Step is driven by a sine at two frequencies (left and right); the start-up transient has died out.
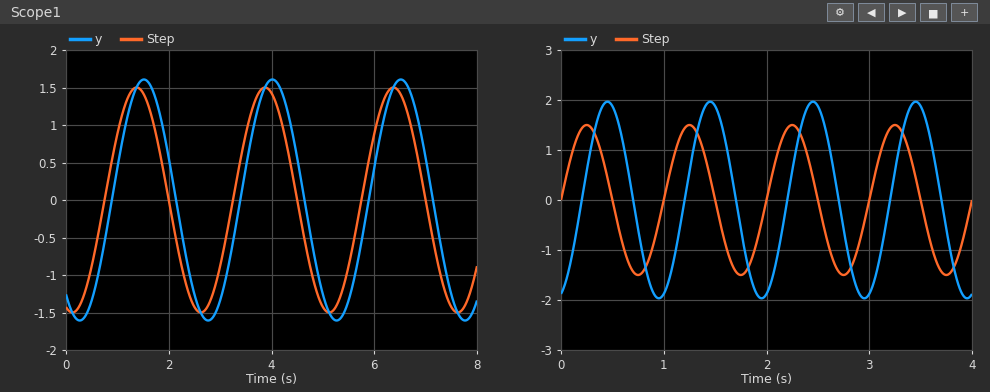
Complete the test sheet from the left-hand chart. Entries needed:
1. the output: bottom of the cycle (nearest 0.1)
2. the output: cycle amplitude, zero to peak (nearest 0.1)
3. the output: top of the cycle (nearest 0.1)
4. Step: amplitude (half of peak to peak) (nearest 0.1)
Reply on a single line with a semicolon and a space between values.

-1.6; 1.6; 1.6; 1.5
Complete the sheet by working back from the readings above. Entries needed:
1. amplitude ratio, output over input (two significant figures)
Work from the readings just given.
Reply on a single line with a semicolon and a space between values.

1.1
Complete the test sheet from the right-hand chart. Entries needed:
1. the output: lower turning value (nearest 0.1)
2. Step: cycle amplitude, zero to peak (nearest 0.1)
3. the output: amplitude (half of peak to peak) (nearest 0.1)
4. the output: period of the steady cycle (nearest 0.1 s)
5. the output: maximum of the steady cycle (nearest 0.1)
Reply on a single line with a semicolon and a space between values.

-2.0; 1.5; 2.0; 1.0 s; 2.0
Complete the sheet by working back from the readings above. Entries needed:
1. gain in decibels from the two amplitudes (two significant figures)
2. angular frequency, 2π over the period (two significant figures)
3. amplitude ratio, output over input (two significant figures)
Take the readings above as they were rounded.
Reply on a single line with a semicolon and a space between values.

2.5 dB; 6.3 rad/s; 1.3
